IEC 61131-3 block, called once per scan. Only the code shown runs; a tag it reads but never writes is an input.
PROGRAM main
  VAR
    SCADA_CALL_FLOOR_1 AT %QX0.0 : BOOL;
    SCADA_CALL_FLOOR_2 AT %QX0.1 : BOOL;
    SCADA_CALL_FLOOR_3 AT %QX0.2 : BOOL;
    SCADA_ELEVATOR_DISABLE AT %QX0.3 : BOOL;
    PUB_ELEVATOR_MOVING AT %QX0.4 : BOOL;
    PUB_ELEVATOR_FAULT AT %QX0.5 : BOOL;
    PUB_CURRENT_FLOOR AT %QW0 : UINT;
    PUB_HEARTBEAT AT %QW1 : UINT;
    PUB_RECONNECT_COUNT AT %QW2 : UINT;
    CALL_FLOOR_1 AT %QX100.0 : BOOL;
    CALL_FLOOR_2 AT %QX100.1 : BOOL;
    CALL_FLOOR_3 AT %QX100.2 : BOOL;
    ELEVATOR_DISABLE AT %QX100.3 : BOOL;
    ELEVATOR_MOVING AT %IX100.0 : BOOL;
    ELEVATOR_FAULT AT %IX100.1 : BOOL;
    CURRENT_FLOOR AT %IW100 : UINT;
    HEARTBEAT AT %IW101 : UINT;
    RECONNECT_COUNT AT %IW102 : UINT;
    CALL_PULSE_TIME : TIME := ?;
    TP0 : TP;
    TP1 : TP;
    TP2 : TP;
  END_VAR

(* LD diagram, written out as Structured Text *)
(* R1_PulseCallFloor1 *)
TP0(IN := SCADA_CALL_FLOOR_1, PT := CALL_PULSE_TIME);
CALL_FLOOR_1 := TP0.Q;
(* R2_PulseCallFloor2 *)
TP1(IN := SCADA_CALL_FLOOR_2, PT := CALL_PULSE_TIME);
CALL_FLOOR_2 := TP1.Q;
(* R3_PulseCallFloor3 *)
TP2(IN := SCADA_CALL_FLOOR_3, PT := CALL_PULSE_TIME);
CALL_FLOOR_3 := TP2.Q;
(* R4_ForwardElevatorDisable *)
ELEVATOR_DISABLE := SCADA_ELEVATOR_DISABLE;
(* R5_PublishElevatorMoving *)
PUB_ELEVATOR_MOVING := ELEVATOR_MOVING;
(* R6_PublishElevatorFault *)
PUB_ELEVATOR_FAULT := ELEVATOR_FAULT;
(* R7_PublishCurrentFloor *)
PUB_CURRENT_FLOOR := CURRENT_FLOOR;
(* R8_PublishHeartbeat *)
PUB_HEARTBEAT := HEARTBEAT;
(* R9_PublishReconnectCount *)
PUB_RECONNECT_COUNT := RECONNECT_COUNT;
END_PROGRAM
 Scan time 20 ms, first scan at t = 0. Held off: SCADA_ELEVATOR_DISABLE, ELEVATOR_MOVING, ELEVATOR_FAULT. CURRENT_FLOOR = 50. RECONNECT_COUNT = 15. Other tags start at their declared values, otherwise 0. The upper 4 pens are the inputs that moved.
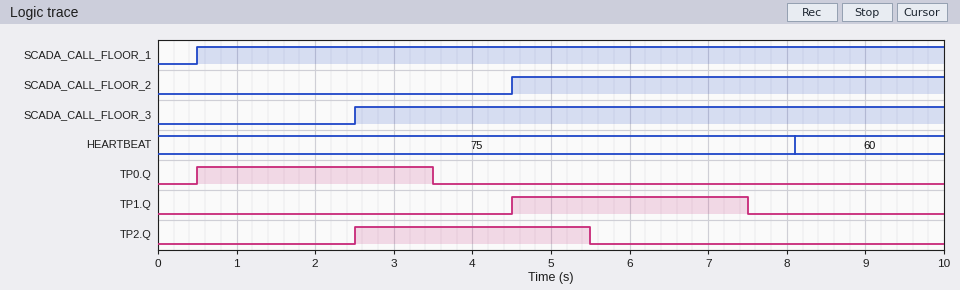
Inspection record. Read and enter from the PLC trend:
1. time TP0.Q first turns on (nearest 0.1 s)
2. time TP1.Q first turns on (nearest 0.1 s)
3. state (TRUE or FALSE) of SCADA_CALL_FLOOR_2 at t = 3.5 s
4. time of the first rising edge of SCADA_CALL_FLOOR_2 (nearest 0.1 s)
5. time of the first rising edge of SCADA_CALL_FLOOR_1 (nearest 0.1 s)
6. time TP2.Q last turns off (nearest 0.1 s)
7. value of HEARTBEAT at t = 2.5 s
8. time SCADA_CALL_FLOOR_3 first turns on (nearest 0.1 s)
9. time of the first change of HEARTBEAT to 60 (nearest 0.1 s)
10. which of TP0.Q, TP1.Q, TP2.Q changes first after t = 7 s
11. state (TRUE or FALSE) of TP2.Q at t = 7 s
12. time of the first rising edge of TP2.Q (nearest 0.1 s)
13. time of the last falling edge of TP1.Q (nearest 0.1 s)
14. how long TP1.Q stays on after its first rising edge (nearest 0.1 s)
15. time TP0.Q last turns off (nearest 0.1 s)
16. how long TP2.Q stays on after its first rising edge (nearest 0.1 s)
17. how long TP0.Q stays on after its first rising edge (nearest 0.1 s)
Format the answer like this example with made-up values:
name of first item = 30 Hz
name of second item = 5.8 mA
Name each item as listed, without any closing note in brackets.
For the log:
time TP0.Q first turns on = 0.5 s
time TP1.Q first turns on = 4.5 s
state (TRUE or FALSE) of SCADA_CALL_FLOOR_2 at t = 3.5 s = FALSE
time of the first rising edge of SCADA_CALL_FLOOR_2 = 4.5 s
time of the first rising edge of SCADA_CALL_FLOOR_1 = 0.5 s
time TP2.Q last turns off = 5.5 s
value of HEARTBEAT at t = 2.5 s = 75
time SCADA_CALL_FLOOR_3 first turns on = 2.5 s
time of the first change of HEARTBEAT to 60 = 8.1 s
which of TP0.Q, TP1.Q, TP2.Q changes first after t = 7 s = TP1.Q
state (TRUE or FALSE) of TP2.Q at t = 7 s = FALSE
time of the first rising edge of TP2.Q = 2.5 s
time of the last falling edge of TP1.Q = 7.5 s
how long TP1.Q stays on after its first rising edge = 3.0 s
time TP0.Q last turns off = 3.5 s
how long TP2.Q stays on after its first rising edge = 3.0 s
how long TP0.Q stays on after its first rising edge = 3.0 s
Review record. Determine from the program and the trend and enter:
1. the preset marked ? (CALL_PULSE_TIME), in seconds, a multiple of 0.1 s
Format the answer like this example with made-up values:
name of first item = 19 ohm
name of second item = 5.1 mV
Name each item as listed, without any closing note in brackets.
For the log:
the preset marked ? (CALL_PULSE_TIME), in seconds, a multiple of 0.1 s = 3.0 s
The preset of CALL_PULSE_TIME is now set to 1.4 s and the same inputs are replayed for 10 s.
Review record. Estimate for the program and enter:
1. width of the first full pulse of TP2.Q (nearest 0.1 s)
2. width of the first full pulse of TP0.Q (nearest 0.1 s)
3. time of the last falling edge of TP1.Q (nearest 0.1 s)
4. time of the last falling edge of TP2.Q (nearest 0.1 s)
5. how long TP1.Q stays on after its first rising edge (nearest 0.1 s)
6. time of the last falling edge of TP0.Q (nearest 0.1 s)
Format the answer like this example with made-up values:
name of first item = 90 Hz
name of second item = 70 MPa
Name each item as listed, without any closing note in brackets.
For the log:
width of the first full pulse of TP2.Q = 1.4 s
width of the first full pulse of TP0.Q = 1.4 s
time of the last falling edge of TP1.Q = 5.9 s
time of the last falling edge of TP2.Q = 3.9 s
how long TP1.Q stays on after its first rising edge = 1.4 s
time of the last falling edge of TP0.Q = 1.9 s
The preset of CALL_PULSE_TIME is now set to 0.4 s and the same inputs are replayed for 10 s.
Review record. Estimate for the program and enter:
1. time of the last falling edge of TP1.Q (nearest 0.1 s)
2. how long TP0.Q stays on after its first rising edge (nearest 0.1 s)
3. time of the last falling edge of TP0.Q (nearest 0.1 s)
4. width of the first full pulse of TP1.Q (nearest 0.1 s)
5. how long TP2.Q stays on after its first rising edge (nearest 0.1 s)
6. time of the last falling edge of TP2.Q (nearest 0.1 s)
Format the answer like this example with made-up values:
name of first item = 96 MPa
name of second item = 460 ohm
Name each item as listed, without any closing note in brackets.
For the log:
time of the last falling edge of TP1.Q = 4.9 s
how long TP0.Q stays on after its first rising edge = 0.4 s
time of the last falling edge of TP0.Q = 0.9 s
width of the first full pulse of TP1.Q = 0.4 s
how long TP2.Q stays on after its first rising edge = 0.4 s
time of the last falling edge of TP2.Q = 2.9 s
